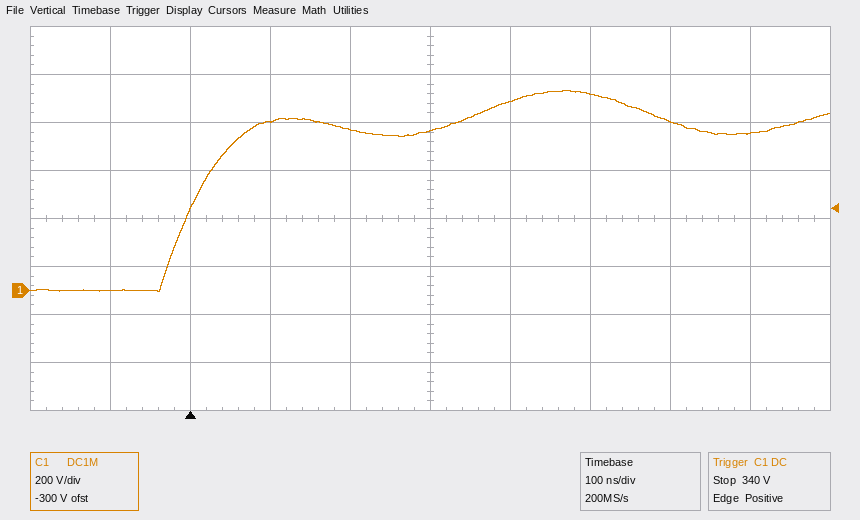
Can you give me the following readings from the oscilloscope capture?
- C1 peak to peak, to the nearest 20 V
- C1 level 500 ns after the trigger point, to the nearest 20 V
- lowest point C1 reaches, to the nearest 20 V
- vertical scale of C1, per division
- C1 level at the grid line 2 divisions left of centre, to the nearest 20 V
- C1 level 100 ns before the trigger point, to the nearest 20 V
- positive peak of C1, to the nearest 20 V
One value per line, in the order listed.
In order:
840 V
820 V
0 V
200 V
700 V
0 V
840 V
